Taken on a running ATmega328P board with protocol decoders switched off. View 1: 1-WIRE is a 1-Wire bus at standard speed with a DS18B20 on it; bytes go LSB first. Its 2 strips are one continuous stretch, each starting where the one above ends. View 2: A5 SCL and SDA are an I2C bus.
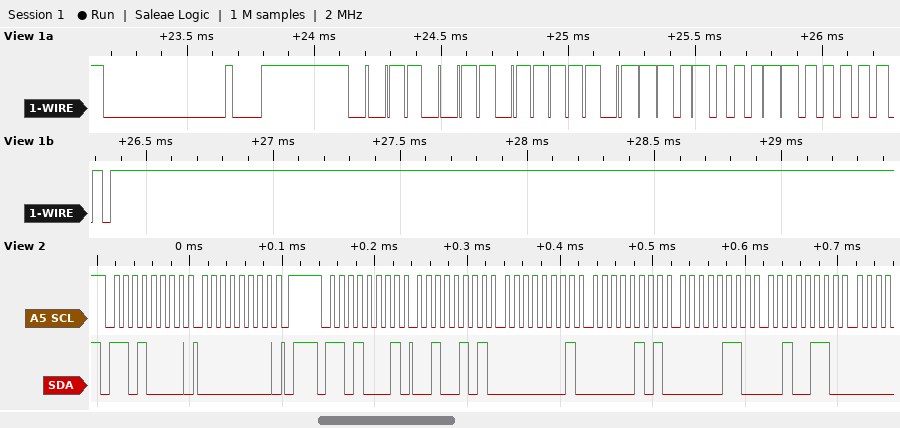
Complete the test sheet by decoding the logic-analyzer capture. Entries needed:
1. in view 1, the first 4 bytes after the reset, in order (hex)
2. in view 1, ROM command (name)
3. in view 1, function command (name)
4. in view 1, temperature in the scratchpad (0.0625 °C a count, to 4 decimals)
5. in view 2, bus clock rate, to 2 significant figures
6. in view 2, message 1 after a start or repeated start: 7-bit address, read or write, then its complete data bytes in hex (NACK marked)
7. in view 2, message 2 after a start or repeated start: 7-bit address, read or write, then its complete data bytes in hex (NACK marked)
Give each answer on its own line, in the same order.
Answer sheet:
CC BE 8B 01
Skip ROM
Read Scratchpad
24.6875 °C
100 kHz
0x68 write: 00
0x68 read: 25 01 05 06 26
